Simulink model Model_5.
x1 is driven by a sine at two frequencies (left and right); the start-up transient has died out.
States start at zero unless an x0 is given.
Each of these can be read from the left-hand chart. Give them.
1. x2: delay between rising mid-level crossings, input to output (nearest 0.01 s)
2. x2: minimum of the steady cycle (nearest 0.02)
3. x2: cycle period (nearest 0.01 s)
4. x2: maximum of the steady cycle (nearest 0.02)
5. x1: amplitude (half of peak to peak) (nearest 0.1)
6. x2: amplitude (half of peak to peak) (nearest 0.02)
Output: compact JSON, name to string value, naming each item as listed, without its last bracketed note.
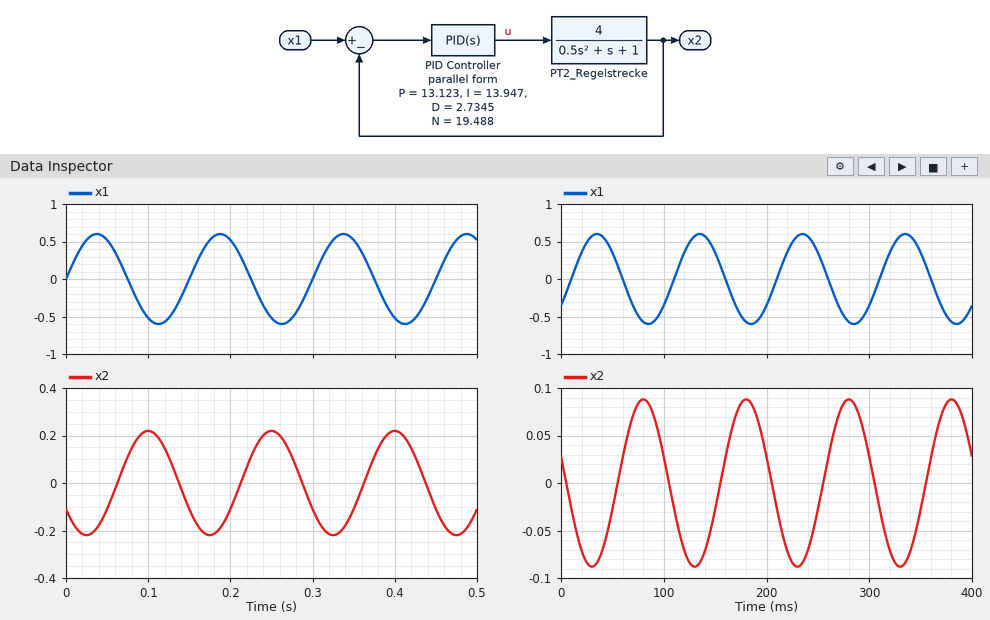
{"x2: delay between rising mid-level crossings, input to output": "0.06 s", "x2: minimum of the steady cycle": "-0.22", "x2: cycle period": "0.15 s", "x2: maximum of the steady cycle": "0.22", "x1: amplitude (half of peak to peak)": "0.6", "x2: amplitude (half of peak to peak)": "0.22"}
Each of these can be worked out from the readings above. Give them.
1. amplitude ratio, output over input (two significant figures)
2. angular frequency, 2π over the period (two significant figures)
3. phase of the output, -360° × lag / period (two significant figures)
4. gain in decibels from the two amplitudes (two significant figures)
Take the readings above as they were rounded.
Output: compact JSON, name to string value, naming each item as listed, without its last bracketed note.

{"amplitude ratio, output over input": "0.37", "angular frequency, 2π over the period": "42 rad/s", "phase of the output, -360° × lag / period": "-140°", "gain in decibels from the two amplitudes": "-8.7 dB"}
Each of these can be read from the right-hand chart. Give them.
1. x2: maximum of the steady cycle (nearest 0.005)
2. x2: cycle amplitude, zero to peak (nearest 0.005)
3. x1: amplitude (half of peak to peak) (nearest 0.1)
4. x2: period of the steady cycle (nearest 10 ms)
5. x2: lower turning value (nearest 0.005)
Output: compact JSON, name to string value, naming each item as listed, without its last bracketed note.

{"x2: maximum of the steady cycle": "0.090", "x2: cycle amplitude, zero to peak": "0.090", "x1: amplitude (half of peak to peak)": "0.6", "x2: period of the steady cycle": "100 ms", "x2: lower turning value": "-0.090"}
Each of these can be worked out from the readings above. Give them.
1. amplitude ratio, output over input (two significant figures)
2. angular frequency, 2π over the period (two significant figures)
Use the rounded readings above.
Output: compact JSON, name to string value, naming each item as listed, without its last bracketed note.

{"amplitude ratio, output over input": "0.15", "angular frequency, 2π over the period": "0.063 rad/ms"}
